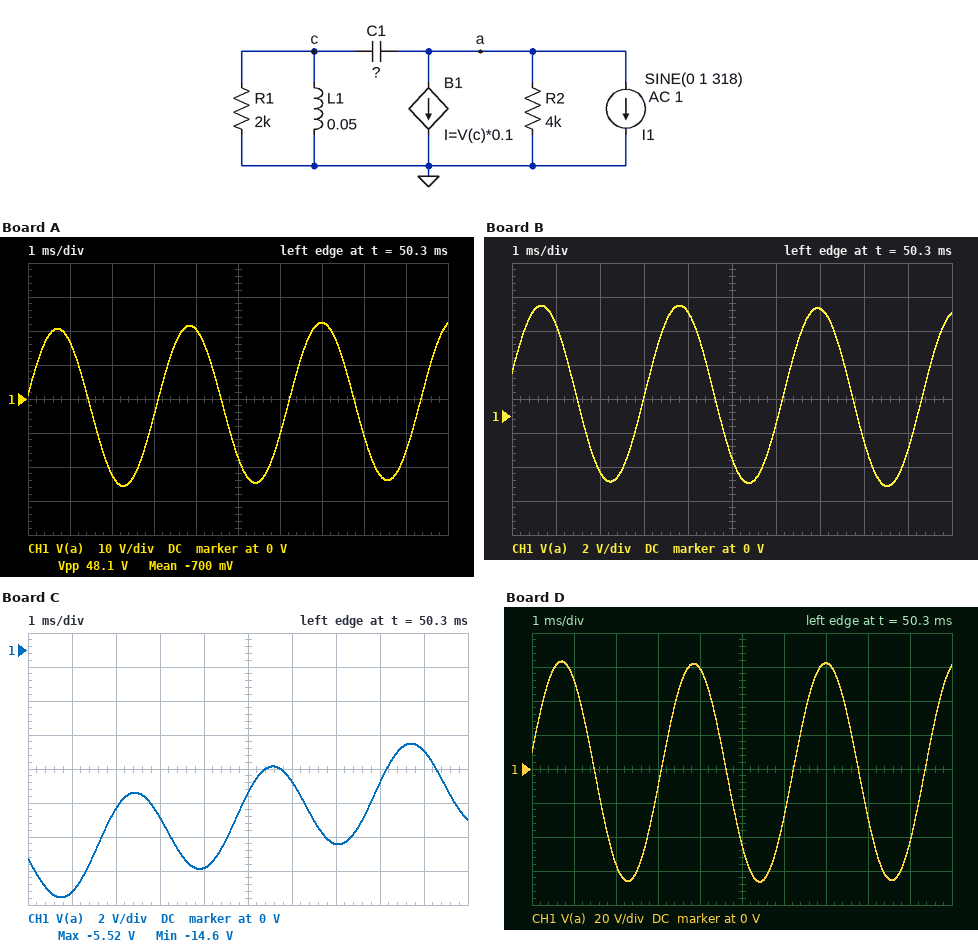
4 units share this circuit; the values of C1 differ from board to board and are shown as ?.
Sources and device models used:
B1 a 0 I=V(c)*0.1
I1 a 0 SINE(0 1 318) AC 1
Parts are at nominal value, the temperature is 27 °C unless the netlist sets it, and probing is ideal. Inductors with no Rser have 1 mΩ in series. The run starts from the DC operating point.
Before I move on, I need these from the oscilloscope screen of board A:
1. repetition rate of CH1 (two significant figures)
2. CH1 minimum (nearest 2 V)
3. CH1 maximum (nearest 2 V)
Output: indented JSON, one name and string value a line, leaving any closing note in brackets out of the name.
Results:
{
  "repetition rate of CH1": "320 Hz",
  "CH1 minimum": "-26 V",
  "CH1 maximum": "22 V"
}
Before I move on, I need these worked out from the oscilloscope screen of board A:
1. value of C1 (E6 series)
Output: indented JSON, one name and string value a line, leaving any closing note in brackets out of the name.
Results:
{
  "value of C1": "1.5 µF"
}
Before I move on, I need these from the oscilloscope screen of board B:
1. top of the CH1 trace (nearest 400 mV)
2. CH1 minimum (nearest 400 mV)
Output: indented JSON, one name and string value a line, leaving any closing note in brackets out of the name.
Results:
{
  "top of the CH1 trace": "6.4 V",
  "CH1 minimum": "-4.0 V"
}
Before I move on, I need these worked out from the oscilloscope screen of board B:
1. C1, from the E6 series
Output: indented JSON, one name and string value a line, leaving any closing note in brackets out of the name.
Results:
{
  "C1, from the E6 series": "3.3 µF"
}
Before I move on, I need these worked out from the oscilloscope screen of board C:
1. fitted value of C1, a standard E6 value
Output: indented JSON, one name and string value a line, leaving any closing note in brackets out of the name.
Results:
{
  "fitted value of C1, a standard E6 value": "6.8 µF"
}
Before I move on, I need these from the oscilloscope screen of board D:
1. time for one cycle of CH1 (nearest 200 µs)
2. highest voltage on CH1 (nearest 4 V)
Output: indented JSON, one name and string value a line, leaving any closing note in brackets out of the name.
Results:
{
  "time for one cycle of CH1": "3.2 ms",
  "highest voltage on CH1": "64 V"
}
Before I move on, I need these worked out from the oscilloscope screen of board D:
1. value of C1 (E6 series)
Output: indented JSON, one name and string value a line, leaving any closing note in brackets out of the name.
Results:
{
  "value of C1": "680 nF"
}
